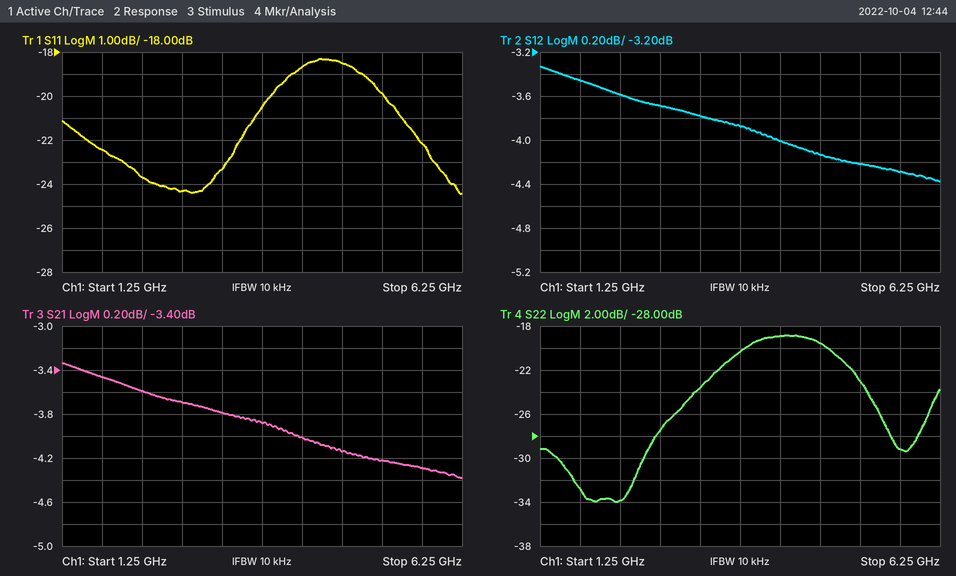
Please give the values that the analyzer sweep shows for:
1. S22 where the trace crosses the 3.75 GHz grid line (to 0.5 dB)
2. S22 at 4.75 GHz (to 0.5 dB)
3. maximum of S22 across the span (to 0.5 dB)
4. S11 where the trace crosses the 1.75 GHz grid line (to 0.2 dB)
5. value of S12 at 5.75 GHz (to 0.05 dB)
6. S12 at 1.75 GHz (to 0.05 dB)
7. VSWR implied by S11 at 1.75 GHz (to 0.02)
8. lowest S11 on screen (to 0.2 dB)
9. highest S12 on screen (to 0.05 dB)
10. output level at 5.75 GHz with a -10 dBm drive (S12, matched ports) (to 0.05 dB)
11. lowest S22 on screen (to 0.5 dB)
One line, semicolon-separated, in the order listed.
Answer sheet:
-20.5 dB; -19.5 dB; -19.0 dB; -22.4 dB; -4.30 dB; -3.45 dB; 1.16; -24.4 dB; -3.35 dB; -14.30 dBm; -34.0 dB
